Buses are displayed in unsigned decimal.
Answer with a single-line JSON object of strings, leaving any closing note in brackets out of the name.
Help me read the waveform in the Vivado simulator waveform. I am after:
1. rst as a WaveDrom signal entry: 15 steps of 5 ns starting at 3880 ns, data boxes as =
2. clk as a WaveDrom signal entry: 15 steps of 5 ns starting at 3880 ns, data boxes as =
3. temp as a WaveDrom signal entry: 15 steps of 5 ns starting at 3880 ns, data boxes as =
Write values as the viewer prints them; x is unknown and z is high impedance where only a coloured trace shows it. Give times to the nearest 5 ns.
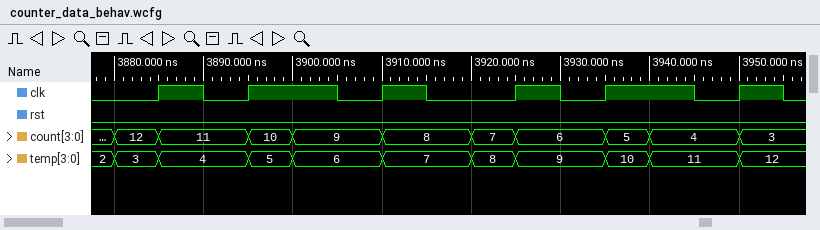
{"rst as a WaveDrom signal entry: 15 steps of 5 ns starting at 3880 ns, data boxes as =": "{name: 'rst', wave: '0..............'}", "clk as a WaveDrom signal entry: 15 steps of 5 ns starting at 3880 ns, data boxes as =": "{name: 'clk', wave: '0101.010.101.01'}", "temp as a WaveDrom signal entry: 15 steps of 5 ns starting at 3880 ns, data boxes as =": "{name: 'temp', wave: '==.==.=.==.==.=', data: '3 4 5 6 7 8 9 10 11 12'}"}
